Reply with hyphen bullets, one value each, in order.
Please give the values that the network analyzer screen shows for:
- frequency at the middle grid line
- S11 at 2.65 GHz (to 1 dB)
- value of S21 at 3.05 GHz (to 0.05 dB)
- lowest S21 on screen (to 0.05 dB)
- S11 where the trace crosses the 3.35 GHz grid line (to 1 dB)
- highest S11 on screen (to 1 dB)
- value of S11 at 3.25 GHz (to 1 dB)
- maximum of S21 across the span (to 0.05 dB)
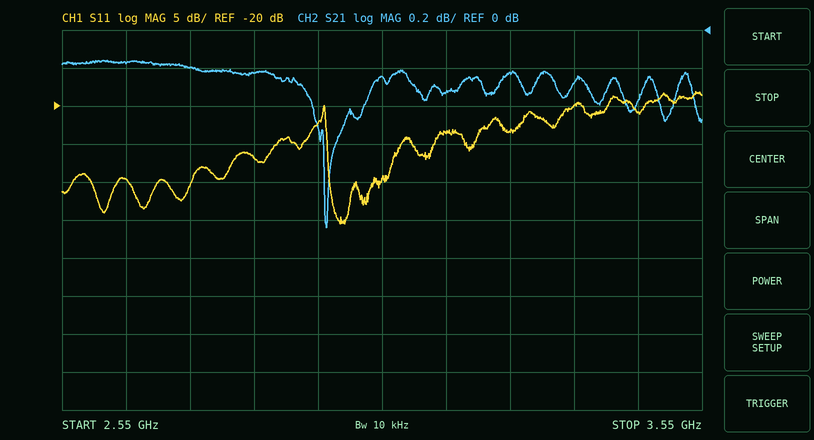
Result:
- 3.05 GHz
- -30 dB
- -0.25 dB
- -1.05 dB
- -20 dB
- -18 dB
- -23 dB
- -0.15 dB
